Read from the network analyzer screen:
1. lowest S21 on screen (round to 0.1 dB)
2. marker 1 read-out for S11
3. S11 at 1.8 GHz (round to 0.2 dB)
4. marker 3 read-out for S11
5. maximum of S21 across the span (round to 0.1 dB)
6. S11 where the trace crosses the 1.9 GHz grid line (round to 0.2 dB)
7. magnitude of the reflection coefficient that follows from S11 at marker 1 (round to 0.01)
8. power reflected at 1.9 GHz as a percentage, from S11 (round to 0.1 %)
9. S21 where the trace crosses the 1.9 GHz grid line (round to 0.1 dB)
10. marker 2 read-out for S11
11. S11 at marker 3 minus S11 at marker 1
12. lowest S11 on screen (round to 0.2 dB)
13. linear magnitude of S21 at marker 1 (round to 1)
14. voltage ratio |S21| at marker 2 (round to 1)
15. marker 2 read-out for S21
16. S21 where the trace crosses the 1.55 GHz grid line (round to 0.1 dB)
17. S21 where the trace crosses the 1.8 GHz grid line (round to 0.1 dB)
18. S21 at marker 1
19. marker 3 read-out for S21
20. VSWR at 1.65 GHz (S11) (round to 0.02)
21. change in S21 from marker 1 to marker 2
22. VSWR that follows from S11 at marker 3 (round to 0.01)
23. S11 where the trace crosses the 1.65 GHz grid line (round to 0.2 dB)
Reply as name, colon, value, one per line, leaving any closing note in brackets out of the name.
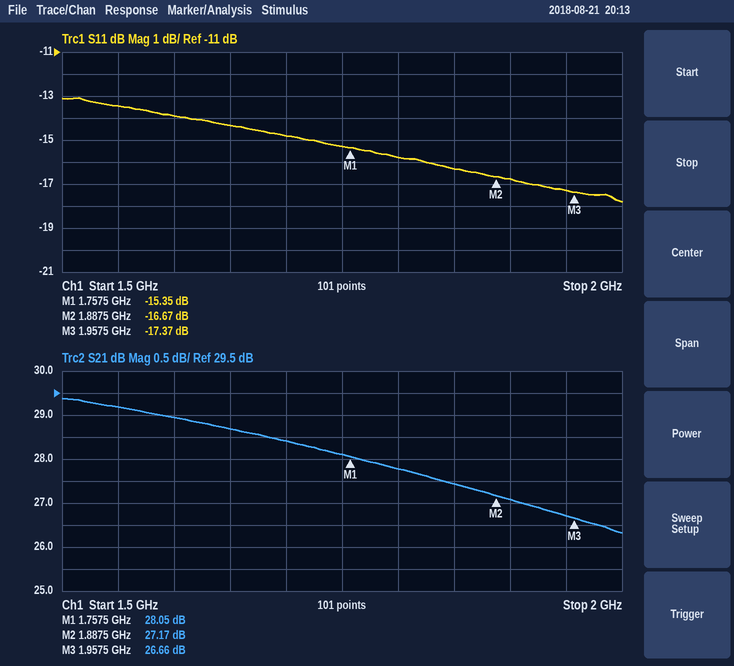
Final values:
lowest S21 on screen: 26.3 dB
marker 1 read-out for S11: -15.35 dB
S11 at 1.8 GHz: -15.8 dB
marker 3 read-out for S11: -17.37 dB
maximum of S21 across the span: 29.4 dB
S11 where the trace crosses the 1.9 GHz grid line: -16.8 dB
magnitude of the reflection coefficient that follows from S11 at marker 1: 0.17
power reflected at 1.9 GHz as a percentage, from S11: 2.1 %
S21 where the trace crosses the 1.9 GHz grid line: 27.1 dB
marker 2 read-out for S11: -16.67 dB
S11 at marker 3 minus S11 at marker 1: -2.02 dB
lowest S11 on screen: -17.8 dB
linear magnitude of S21 at marker 1: 25
voltage ratio |S21| at marker 2: 23
marker 2 read-out for S21: 27.17 dB
S21 where the trace crosses the 1.55 GHz grid line: 29.2 dB
S21 where the trace crosses the 1.8 GHz grid line: 27.8 dB
S21 at marker 1: 28.05 dB
marker 3 read-out for S21: 26.66 dB
VSWR at 1.65 GHz (S11): 1.48
change in S21 from marker 1 to marker 2: -0.88 dB
VSWR that follows from S11 at marker 3: 1.31
S11 where the trace crosses the 1.65 GHz grid line: -14.4 dB
